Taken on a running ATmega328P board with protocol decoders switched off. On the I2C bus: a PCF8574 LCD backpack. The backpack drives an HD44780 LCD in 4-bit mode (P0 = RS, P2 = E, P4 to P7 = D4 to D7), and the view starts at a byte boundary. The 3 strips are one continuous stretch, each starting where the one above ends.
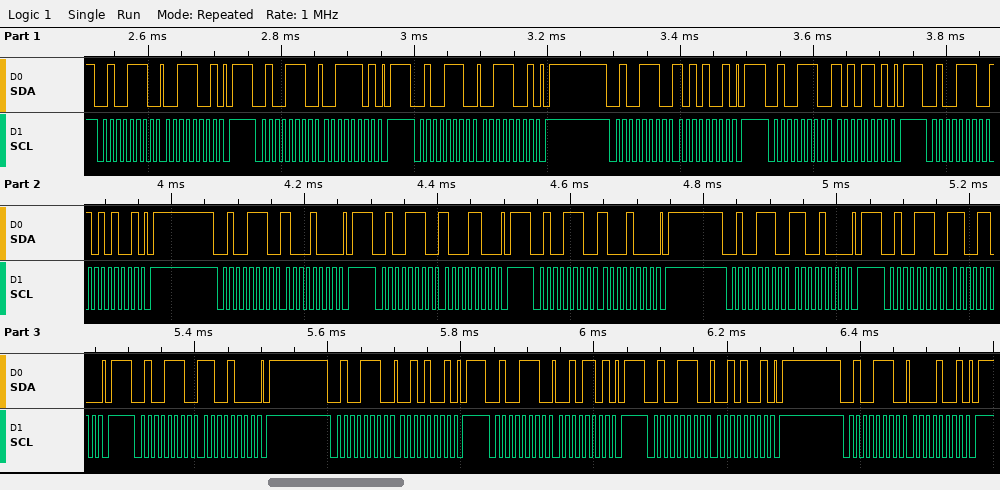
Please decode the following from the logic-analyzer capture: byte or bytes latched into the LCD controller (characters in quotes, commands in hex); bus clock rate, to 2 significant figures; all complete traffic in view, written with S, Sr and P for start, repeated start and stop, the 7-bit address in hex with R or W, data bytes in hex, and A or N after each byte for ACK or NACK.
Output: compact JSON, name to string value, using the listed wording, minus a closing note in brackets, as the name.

{"byte or bytes latched into the LCD controller": "':' 0x8C", "bus clock rate, to 2 significant figures": "100 kHz", "all complete traffic in view, written with S, Sr and P for start, repeated start and stop, the 7-bit address in hex with R or W, data bytes in hex, and A or N after each byte for ACK or NACK": "S 27W A 39 A P S 27W A 3D A P S 27W A 39 A P S 27W A A9 A P S 27W A AD A P S 27W A A9 A P S 27W A 88 A P S 27W A 8C A P S 27W A 88 A P S 27W A C8 A P S 27W A CC A P S 27W A C8 A P S 27W A 29 A P S 27W A 2D A P S 27W A 29 A P S 27W A 09 A P"}
